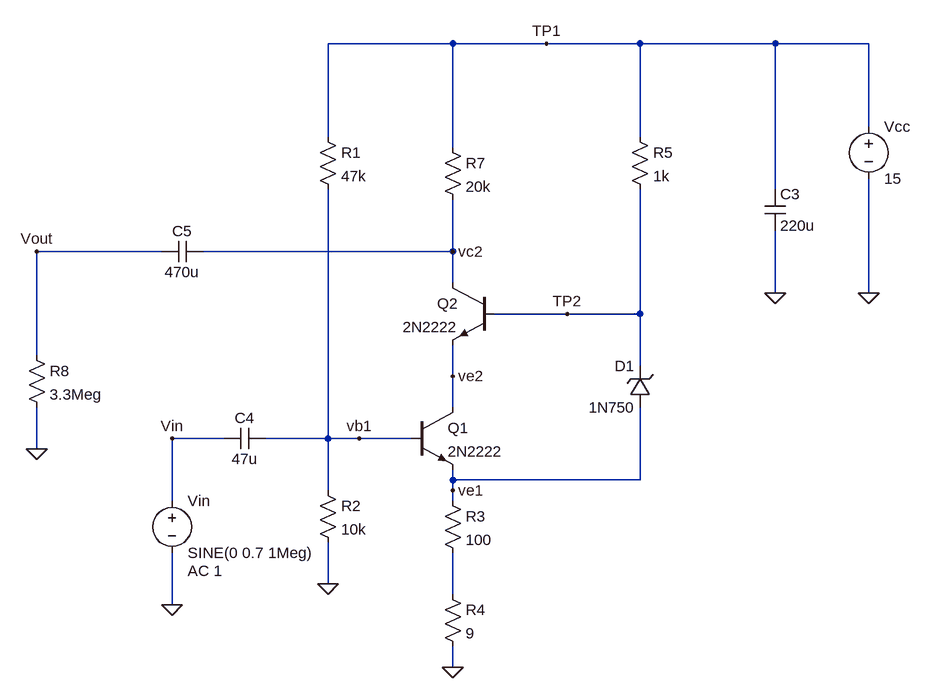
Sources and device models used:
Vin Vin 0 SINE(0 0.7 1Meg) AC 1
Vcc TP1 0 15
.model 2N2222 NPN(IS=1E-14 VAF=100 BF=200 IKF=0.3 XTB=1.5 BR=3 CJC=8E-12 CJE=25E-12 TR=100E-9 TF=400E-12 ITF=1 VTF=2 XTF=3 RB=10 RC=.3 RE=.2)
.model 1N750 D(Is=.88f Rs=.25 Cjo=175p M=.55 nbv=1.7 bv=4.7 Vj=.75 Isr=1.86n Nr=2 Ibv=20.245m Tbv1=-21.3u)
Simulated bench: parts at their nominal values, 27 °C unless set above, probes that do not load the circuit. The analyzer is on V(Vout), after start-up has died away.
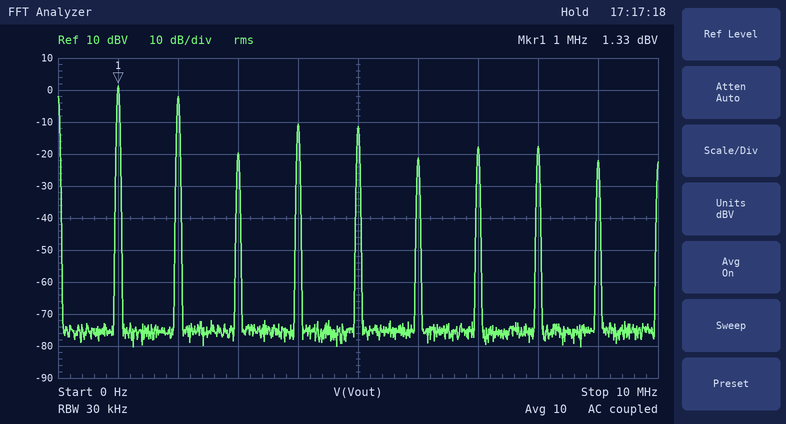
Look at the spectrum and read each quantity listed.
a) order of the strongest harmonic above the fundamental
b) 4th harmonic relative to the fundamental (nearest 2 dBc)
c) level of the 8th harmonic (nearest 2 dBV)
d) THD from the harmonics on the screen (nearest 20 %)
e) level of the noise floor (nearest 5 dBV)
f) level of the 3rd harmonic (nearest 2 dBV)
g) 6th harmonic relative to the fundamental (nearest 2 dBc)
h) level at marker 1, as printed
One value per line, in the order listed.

2
-12 dBc
-18 dBV
80 %
-75 dBV
-20 dBV
-22 dBc
1.33 dBV
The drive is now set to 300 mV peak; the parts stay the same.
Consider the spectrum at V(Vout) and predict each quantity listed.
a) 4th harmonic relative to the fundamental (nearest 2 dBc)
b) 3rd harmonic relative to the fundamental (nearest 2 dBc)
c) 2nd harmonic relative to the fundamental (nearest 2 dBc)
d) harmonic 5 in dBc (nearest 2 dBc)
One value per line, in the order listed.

-16 dBc
-18 dBc
-6 dBc
-20 dBc
